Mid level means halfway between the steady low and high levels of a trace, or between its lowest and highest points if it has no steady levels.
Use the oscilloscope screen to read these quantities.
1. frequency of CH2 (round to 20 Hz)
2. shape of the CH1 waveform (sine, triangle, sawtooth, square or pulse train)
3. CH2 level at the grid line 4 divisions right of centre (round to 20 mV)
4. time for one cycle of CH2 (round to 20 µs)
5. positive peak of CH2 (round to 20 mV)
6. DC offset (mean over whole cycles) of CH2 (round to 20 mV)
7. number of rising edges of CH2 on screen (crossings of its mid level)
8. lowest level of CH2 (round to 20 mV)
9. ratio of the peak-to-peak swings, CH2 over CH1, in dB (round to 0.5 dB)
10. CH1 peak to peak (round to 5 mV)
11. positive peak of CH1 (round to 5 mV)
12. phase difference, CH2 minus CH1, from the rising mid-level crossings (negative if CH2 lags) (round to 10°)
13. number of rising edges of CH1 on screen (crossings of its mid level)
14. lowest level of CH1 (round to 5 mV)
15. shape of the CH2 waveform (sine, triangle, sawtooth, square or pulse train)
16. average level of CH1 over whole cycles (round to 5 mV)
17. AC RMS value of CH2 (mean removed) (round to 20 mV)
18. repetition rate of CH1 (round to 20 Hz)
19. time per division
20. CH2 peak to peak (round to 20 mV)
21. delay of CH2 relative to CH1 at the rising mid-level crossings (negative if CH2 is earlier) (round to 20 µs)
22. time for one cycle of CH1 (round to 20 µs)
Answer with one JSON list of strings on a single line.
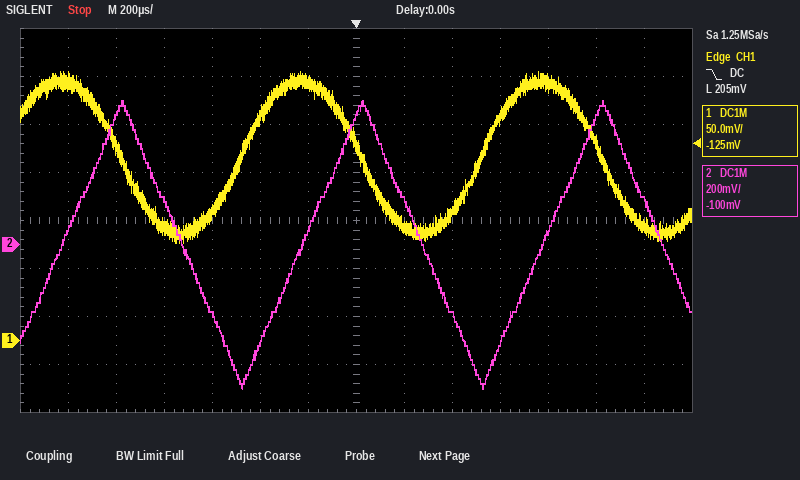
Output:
["1.00 kHz", "sine", "60 mV", "1.00 ms", "600 mV", "0 mV", "3", "-600 mV", "16.5 dB", "180 mV", "280 mV", "-90°", "2", "100 mV", "triangle", "190 mV", "340 mV", "1.00 kHz", "200 µs", "1.20 V", "+260 µs", "1.00 ms"]
